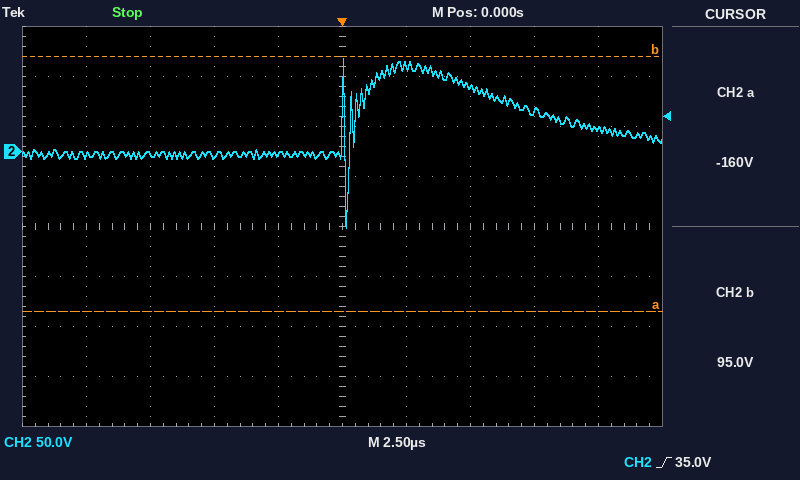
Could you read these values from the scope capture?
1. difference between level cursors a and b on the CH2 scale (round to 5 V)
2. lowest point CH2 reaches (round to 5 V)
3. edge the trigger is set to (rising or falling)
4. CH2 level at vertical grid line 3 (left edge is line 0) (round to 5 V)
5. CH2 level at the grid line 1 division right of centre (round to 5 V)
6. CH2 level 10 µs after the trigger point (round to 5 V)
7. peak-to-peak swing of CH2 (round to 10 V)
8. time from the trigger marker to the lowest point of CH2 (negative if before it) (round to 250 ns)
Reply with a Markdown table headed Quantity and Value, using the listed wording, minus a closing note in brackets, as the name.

| Quantity | Value |
|---|---|
| difference between level cursors a and b on the CH2 scale | 255 V |
| lowest point CH2 reaches | -75 V |
| edge the trigger is set to | rising |
| CH2 level at vertical grid line 3 (left edge is line 0) | -5 V |
| CH2 level at the grid line 1 division right of centre | 85 V |
| CH2 level 10 µs after the trigger point | 25 V |
| peak-to-peak swing of CH2 | 170 V |
| time from the trigger marker to the lowest point of CH2 (negative if before it) | +250 ns |
